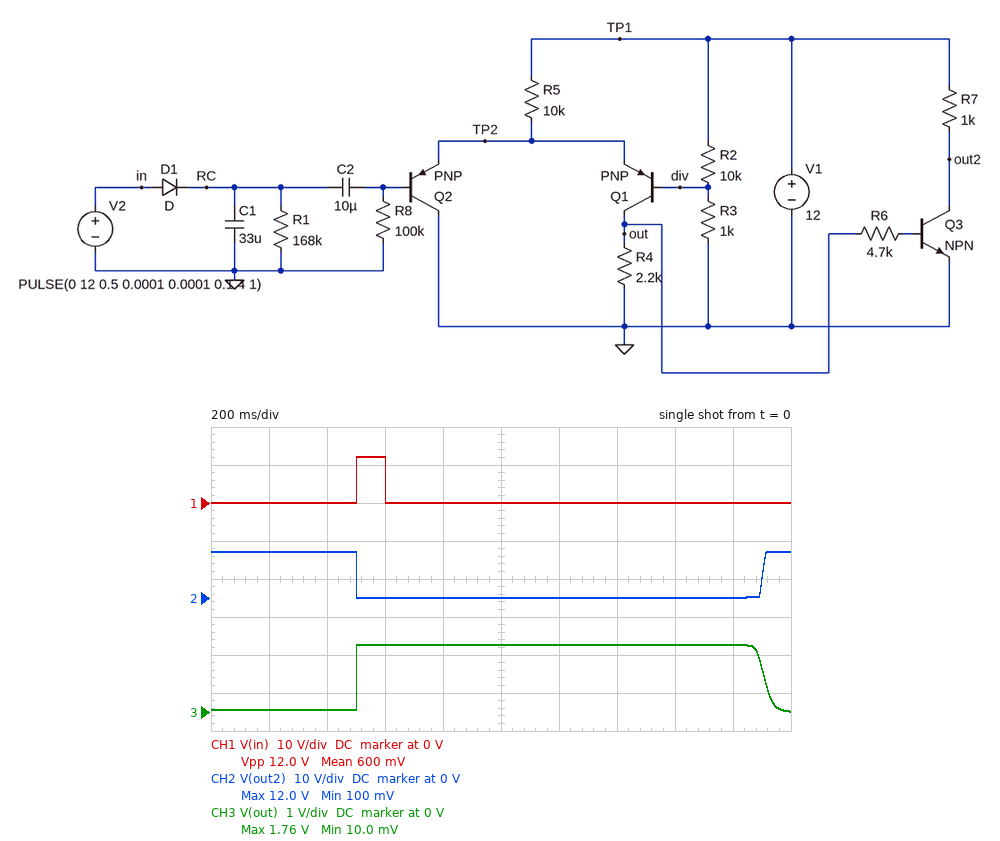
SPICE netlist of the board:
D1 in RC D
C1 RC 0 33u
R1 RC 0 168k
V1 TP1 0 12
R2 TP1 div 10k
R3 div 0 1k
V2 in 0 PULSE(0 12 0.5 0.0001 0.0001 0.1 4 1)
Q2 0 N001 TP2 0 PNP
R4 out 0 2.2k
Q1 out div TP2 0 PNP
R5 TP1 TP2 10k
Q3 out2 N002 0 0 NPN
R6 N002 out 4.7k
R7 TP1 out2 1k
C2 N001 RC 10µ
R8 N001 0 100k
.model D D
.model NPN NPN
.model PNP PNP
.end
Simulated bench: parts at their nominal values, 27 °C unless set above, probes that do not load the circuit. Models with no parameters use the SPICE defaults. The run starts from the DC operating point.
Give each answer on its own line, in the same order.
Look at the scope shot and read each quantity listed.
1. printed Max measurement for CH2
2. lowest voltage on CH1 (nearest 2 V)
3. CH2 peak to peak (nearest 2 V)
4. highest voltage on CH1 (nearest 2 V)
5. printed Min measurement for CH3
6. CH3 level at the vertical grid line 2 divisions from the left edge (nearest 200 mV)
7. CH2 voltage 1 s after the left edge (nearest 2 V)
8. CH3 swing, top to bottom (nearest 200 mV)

12.0 V
0 V
12 V
12 V
10.0 mV
0 V
0 V
1.8 V
